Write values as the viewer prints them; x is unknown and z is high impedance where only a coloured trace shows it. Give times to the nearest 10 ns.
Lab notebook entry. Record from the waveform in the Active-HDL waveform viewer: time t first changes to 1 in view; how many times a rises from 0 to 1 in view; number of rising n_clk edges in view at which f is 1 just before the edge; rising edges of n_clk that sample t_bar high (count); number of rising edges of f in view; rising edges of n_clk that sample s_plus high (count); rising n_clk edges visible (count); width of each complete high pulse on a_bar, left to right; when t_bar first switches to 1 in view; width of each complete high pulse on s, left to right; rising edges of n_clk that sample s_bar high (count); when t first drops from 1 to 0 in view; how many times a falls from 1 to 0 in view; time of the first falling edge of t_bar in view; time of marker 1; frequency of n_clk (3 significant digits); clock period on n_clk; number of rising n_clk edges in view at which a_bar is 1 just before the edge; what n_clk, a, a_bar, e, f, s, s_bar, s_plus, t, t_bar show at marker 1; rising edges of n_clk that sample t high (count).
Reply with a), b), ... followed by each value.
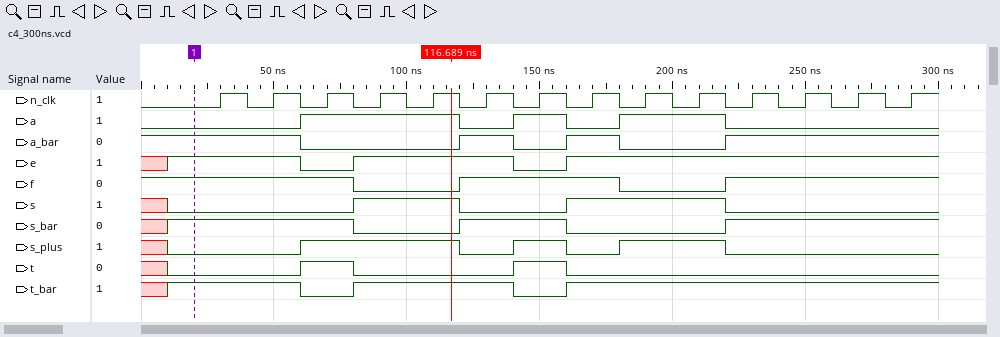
a) 60 ns
b) 3
c) 10
d) 12
e) 2
f) 6
g) 14
h) 20 ns, 20 ns
i) 10 ns
j) 40 ns, 60 ns
k) 9
l) 80 ns
m) 3
n) 60 ns
o) 20 ns
p) 50.0 MHz
q) 20 ns
r) 8
s) n_clk=0, a=0, a_bar=1, e=1, f=1, s=0, s_bar=1, s_plus=0, t=0, t_bar=1
t) 2
